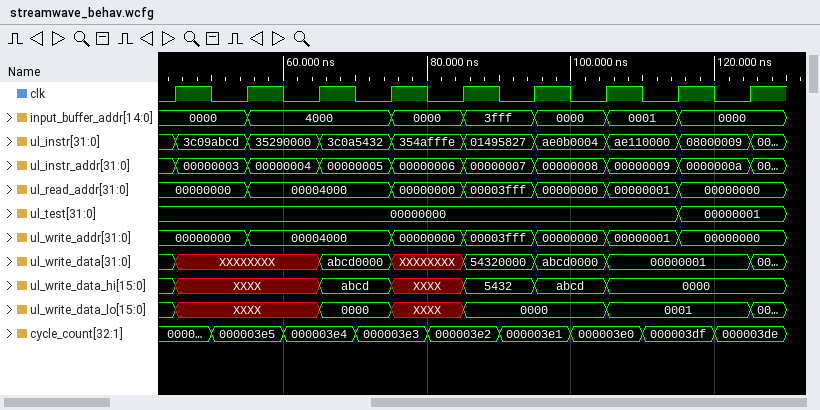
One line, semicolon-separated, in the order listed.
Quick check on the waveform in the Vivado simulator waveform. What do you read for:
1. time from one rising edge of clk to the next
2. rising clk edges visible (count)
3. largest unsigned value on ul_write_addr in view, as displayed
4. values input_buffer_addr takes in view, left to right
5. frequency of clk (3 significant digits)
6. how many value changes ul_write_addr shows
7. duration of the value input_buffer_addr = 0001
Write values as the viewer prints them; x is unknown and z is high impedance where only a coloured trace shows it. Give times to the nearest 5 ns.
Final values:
10 ns; 9; 00004000; 0000, 4000, 0000, 3fff, 0000, 0001, 0000; 100 MHz; 6; 10 ns
